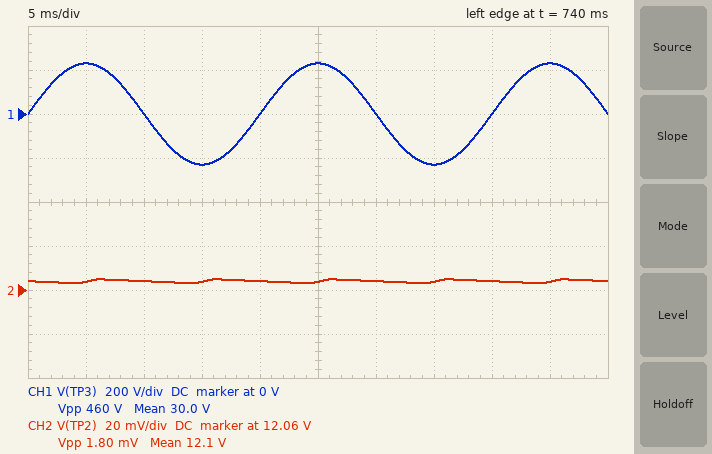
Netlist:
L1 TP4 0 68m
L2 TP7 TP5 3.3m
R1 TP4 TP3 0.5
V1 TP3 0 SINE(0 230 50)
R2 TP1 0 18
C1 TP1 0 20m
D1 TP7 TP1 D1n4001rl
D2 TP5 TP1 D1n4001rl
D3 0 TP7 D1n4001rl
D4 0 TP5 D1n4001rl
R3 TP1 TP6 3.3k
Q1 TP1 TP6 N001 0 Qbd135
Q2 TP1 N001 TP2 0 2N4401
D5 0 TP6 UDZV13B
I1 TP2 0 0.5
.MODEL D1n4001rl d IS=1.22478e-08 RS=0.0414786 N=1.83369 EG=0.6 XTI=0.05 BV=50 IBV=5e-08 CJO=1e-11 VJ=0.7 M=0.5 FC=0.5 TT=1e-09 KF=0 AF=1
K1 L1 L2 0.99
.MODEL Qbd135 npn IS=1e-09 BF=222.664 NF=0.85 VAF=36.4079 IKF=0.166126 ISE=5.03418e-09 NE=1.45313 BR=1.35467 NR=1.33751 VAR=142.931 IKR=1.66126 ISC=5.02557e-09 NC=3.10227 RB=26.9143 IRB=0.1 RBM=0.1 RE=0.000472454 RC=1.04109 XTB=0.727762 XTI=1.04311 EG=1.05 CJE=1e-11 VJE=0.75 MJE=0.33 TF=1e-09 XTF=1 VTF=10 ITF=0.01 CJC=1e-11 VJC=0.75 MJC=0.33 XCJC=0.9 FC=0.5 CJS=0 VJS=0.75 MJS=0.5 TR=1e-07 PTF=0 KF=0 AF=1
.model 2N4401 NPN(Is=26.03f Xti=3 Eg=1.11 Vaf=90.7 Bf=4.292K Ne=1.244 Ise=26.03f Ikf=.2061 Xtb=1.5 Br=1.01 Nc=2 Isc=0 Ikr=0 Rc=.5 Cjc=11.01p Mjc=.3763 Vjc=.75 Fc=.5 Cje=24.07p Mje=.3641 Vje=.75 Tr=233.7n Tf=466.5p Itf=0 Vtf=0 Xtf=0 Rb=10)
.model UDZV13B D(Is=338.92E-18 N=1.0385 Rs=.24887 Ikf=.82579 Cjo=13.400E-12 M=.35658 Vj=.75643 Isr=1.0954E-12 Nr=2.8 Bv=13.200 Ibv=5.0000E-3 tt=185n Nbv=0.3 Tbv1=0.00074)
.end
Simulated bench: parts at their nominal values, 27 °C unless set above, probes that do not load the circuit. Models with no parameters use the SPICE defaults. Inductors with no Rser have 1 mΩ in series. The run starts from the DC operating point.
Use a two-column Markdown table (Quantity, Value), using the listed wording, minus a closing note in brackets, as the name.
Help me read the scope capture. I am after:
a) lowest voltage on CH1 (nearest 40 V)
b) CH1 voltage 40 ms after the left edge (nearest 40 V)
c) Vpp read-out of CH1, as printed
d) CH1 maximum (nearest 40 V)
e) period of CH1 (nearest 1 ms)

| Quantity | Value |
|---|---|
| lowest voltage on CH1 | -240 V |
| CH1 voltage 40 ms after the left edge | 0 V |
| Vpp read-out of CH1, as printed | 460 V |
| CH1 maximum | 240 V |
| period of CH1 | 20 ms |
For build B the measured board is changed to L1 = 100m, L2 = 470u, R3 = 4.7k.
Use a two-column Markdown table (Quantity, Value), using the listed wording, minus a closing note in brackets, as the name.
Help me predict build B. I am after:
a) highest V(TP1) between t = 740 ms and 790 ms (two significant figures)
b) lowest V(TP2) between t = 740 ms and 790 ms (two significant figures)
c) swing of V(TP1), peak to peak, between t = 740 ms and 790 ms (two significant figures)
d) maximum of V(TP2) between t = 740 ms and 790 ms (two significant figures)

| Quantity | Value |
|---|---|
| highest V(TP1) between t = 740 ms and 790 ms | 13 V |
| lowest V(TP2) between t = 740 ms and 790 ms | 11 V |
| swing of V(TP1), peak to peak, between t = 740 ms and 790 ms | 480 mV |
| maximum of V(TP2) between t = 740 ms and 790 ms | 12 V |
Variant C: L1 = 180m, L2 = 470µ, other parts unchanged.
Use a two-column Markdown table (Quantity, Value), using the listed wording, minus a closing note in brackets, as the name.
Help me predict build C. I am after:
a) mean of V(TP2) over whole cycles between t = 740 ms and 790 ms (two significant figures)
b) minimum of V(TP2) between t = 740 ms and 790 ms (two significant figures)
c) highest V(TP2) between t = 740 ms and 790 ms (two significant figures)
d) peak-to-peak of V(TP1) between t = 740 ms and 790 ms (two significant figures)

| Quantity | Value |
|---|---|
| mean of V(TP2) over whole cycles between t = 740 ms and 790 ms | 7.8 V |
| minimum of V(TP2) between t = 740 ms and 790 ms | 7.6 V |
| highest V(TP2) between t = 740 ms and 790 ms | 8.0 V |
| peak-to-peak of V(TP1) between t = 740 ms and 790 ms | 400 mV |
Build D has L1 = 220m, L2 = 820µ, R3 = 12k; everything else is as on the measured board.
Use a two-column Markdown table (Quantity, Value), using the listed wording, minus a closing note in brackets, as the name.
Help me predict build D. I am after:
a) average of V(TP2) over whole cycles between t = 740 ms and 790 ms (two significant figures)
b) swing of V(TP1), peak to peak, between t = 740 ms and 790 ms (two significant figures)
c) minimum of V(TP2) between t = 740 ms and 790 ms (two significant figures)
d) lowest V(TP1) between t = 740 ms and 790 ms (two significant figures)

| Quantity | Value |
|---|---|
| average of V(TP2) over whole cycles between t = 740 ms and 790 ms | 9.5 V |
| swing of V(TP1), peak to peak, between t = 740 ms and 790 ms | 450 mV |
| minimum of V(TP2) between t = 740 ms and 790 ms | 9.3 V |
| lowest V(TP1) between t = 740 ms and 790 ms | 11 V |
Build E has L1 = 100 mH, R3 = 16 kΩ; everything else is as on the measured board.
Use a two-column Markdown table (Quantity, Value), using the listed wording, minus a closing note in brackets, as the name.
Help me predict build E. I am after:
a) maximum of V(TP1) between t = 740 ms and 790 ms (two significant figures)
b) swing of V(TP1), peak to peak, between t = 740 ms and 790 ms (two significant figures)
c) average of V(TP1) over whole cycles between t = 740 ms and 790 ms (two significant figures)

| Quantity | Value |
|---|---|
| maximum of V(TP1) between t = 740 ms and 790 ms | 38 V |
| swing of V(TP1), peak to peak, between t = 740 ms and 790 ms | 1.0 V |
| average of V(TP1) over whole cycles between t = 740 ms and 790 ms | 37 V |
